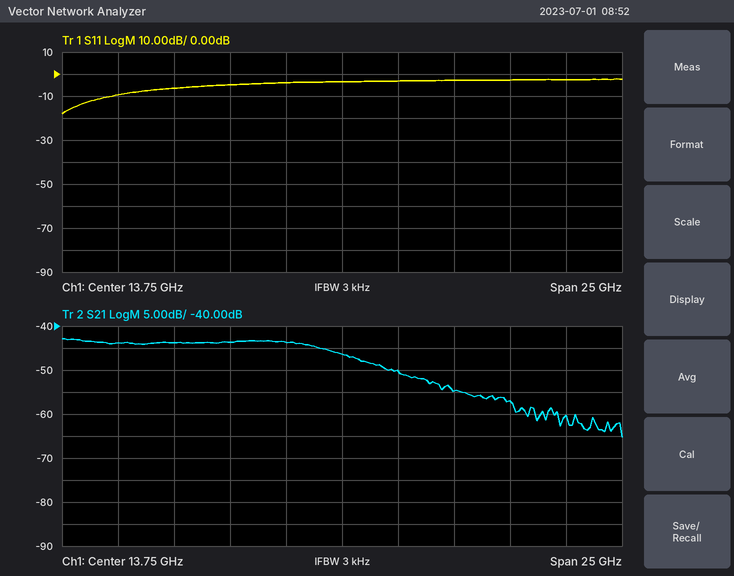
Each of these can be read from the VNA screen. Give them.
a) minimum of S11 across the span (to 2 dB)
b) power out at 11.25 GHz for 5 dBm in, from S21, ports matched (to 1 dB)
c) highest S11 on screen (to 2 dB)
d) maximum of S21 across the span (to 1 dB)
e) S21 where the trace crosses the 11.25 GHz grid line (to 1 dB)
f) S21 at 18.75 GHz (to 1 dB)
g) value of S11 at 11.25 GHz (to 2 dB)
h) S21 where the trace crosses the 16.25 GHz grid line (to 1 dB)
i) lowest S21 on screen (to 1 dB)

-18 dB
-39 dBm
-2 dB
-43 dB
-44 dB
-55 dB
-4 dB
-50 dB
-65 dB
